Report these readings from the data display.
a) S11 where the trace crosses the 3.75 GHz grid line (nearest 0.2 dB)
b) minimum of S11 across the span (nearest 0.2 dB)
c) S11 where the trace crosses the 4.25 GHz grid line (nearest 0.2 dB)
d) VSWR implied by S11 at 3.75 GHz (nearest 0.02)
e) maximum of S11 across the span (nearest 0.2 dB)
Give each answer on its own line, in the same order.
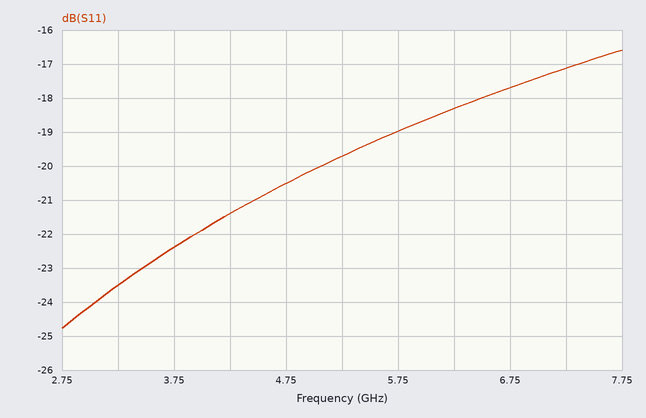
-22.4 dB
-24.8 dB
-21.4 dB
1.16
-16.6 dB
